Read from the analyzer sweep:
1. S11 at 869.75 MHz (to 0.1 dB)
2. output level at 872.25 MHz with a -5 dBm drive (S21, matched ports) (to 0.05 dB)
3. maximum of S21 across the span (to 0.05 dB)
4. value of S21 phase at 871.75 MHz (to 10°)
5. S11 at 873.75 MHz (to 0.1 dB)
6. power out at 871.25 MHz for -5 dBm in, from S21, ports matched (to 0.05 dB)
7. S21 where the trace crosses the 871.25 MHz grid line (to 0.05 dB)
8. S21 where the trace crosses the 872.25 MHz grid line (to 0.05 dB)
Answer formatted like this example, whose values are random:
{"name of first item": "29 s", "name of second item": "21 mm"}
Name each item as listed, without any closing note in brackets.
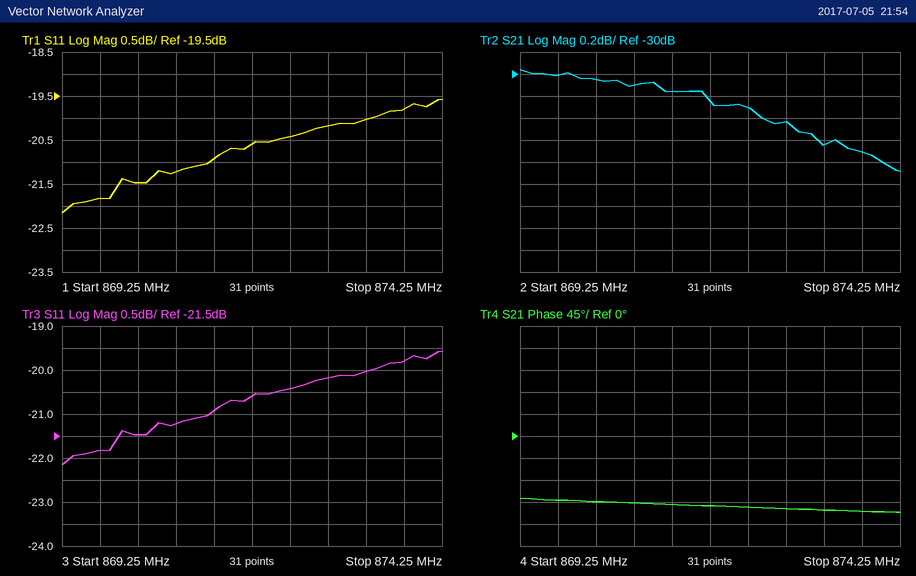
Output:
{"S11 at 869.75 MHz": "-21.8 dB", "output level at 872.25 MHz with a -5 dBm drive (S21, matched ports)": "-35.30 dBm", "maximum of S21 across the span": "-29.95 dB", "value of S21 phase at 871.75 MHz": "-140°", "S11 at 873.75 MHz": "-19.8 dB", "power out at 871.25 MHz for -5 dBm in, from S21, ports matched": "-35.15 dBm", "S21 where the trace crosses the 871.25 MHz grid line": "-30.15 dB", "S21 where the trace crosses the 872.25 MHz grid line": "-30.30 dB"}
